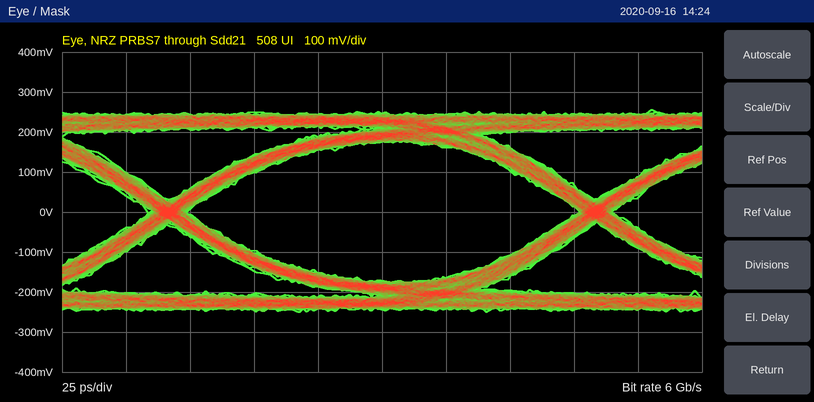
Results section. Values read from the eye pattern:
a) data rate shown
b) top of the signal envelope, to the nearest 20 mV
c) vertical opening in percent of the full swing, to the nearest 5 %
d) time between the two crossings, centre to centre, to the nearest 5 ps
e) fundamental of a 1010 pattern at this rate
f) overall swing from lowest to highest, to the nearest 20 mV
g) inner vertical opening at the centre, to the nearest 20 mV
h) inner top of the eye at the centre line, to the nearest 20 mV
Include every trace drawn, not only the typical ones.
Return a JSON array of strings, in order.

["6 Gb/s", "260 mV", "70 %", "165 ps", "3 GHz", "500 mV", "340 mV", "180 mV"]
